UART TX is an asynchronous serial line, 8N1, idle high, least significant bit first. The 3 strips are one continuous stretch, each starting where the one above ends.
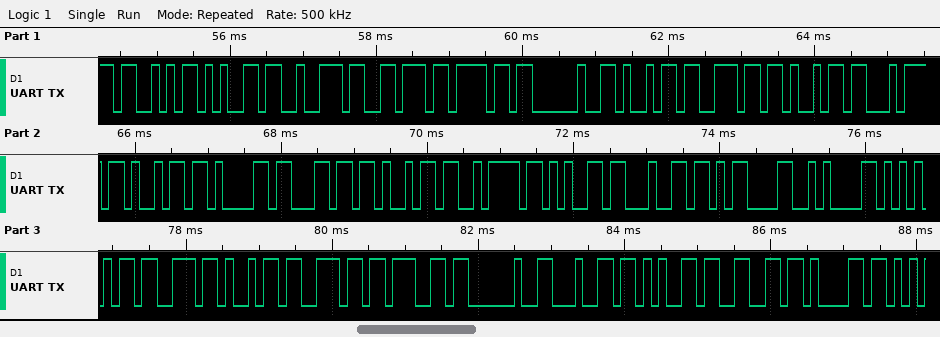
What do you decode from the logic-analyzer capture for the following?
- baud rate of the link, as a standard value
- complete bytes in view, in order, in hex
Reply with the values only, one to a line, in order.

9600 baud
53 65 72 76 6F 20 69 6E 69 74 69 61 6C 69 7A 65 64 0D 0A 55 73 69 6E 67 20 64 65 66 61
